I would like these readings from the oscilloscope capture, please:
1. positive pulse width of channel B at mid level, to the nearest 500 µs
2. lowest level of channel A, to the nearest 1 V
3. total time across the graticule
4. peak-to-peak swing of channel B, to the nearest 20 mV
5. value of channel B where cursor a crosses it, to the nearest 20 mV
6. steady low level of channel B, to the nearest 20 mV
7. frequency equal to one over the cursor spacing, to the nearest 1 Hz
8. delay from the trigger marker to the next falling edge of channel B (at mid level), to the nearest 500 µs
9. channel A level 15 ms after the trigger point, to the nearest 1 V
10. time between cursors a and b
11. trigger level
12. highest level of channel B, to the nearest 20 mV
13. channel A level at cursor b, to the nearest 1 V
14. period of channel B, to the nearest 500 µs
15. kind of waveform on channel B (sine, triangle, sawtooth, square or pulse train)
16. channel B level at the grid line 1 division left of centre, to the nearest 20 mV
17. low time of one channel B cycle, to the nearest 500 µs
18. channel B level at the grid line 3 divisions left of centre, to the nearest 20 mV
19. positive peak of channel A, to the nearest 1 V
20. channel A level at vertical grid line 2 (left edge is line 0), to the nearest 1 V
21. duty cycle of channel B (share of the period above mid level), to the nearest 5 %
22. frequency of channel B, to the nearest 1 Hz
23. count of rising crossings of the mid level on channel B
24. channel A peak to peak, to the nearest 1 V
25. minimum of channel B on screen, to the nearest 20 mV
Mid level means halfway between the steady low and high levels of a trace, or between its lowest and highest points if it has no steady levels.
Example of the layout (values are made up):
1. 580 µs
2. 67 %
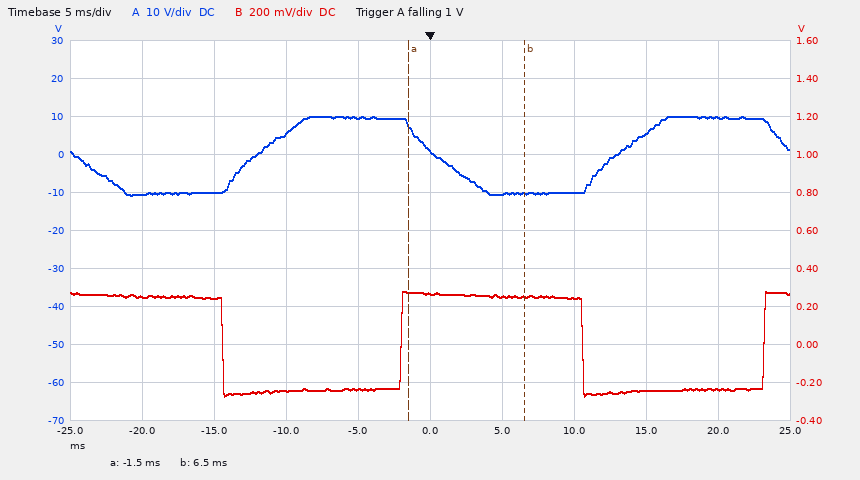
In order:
1. 12.5 ms
2. -11 V
3. 50 ms
4. 560 mV
5. 280 mV
6. -240 mV
7. 125 Hz
8. 10.5 ms
9. 6 V
10. 8.0 ms
11. 1 V
12. 280 mV
13. -10 V
14. 25.0 ms
15. square
16. -240 mV
17. 12.5 ms
18. 240 mV
19. 10 V
20. -10 V
21. 50 %
22. 40 Hz
23. 2
24. 21 V
25. -280 mV
